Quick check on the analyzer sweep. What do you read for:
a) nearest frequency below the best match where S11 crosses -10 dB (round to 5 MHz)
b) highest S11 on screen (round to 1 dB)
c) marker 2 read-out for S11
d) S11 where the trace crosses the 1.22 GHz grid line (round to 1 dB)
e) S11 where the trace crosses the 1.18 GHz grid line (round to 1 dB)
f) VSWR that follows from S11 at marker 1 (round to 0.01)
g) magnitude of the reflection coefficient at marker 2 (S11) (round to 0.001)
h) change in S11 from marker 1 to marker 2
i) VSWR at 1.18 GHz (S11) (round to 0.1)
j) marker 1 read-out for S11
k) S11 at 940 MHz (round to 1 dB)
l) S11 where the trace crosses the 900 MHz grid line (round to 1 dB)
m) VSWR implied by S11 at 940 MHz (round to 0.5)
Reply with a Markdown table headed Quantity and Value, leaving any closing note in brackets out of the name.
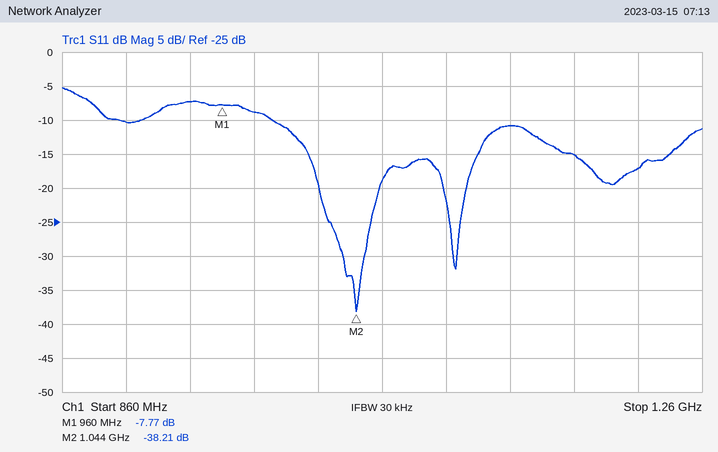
| Quantity | Value |
|---|---|
| nearest frequency below the best match where S11 crosses -10 dB | 990 MHz |
| highest S11 on screen | -5 dB |
| marker 2 read-out for S11 | -38.21 dB |
| S11 where the trace crosses the 1.22 GHz grid line | -17 dB |
| S11 where the trace crosses the 1.18 GHz grid line | -15 dB |
| VSWR that follows from S11 at marker 1 | 2.38 |
| magnitude of the reflection coefficient at marker 2 (S11) | 0.012 |
| change in S11 from marker 1 to marker 2 | -30.44 dB |
| VSWR at 1.18 GHz (S11) | 1.4 |
| marker 1 read-out for S11 | -7.77 dB |
| S11 at 940 MHz | -7 dB |
| S11 where the trace crosses the 900 MHz grid line | -10 dB |
| VSWR implied by S11 at 940 MHz | 2.5 |
